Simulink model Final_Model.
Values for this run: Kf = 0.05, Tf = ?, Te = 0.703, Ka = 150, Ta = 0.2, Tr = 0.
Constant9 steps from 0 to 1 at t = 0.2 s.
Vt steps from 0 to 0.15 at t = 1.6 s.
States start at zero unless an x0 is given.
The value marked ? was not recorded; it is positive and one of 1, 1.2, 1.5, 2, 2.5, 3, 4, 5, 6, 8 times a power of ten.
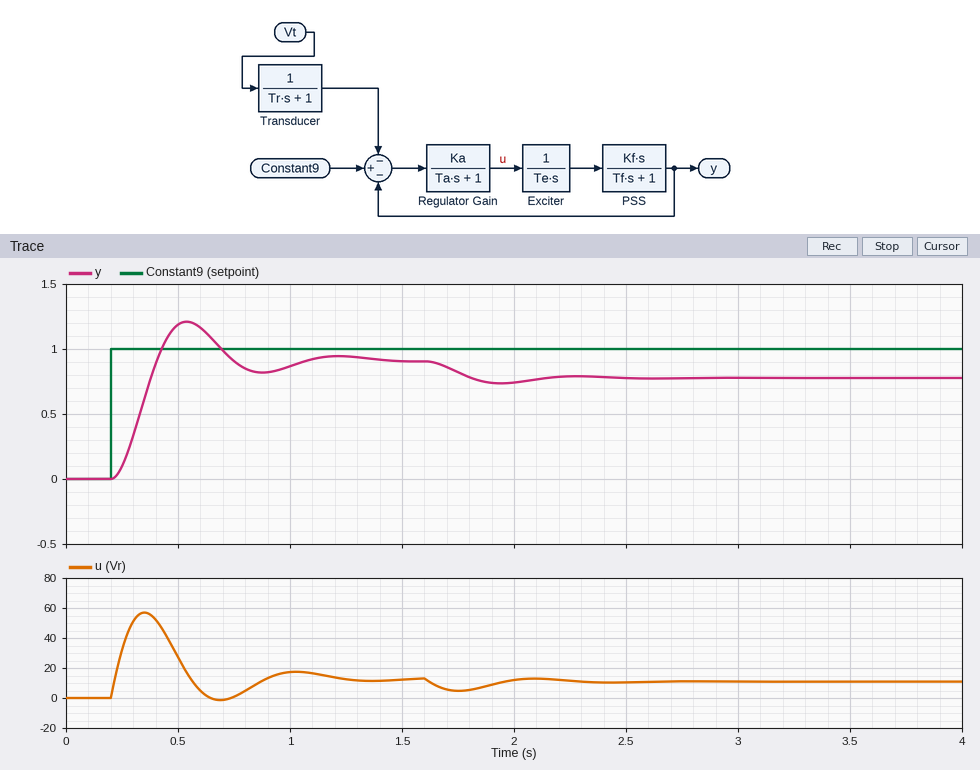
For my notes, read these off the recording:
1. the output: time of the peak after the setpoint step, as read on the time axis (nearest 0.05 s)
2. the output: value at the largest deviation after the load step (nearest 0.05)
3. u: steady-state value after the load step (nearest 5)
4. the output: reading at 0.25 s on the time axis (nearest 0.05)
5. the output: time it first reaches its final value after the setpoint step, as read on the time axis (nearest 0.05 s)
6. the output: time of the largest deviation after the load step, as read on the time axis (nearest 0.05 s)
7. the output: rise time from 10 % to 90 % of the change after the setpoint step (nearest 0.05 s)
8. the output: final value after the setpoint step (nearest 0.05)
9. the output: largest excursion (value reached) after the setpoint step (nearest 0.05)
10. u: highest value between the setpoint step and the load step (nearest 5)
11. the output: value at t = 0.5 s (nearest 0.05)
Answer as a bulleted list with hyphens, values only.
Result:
- 0.55 s
- 0.75
- 10
- 0.10
- 0.40 s
- 1.95 s
- 0.15 s
- 0.90
- 1.20
- 55
- 1.20
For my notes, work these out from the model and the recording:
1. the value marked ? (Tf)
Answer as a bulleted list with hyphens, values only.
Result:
- 0.6
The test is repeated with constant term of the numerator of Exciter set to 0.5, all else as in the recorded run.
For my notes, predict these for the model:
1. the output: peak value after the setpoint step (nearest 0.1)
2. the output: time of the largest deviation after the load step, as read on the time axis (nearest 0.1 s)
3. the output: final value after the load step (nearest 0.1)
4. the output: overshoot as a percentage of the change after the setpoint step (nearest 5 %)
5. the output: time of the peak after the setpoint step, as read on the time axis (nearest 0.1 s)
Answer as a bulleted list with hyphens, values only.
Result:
- 1.0
- 2.1 s
- 0.7
- 20 %
- 0.7 s
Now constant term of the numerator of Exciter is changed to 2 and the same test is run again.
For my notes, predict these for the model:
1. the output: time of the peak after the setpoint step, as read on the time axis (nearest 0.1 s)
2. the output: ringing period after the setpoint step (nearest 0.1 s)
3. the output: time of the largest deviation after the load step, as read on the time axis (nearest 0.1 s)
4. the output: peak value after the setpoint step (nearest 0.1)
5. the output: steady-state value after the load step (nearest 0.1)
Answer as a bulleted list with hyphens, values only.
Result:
- 0.4 s
- 0.5 s
- 1.8 s
- 1.4
- 0.8
